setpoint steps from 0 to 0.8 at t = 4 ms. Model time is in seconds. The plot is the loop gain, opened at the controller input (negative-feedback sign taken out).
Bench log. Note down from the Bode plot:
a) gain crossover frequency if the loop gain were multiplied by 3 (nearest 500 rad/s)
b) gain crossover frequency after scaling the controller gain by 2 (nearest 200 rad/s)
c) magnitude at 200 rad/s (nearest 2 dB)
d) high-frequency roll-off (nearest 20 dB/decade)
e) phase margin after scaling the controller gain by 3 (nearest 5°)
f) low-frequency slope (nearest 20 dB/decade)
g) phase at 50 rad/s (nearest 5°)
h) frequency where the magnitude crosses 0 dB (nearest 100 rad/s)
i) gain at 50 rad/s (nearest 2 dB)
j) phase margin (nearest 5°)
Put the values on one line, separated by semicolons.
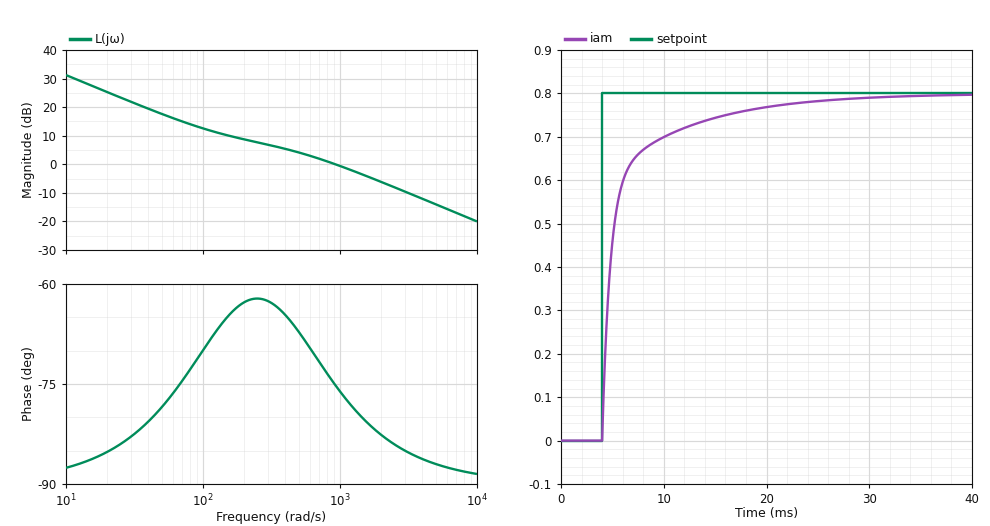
3000 rad/s; 2000 rad/s; 8 dB; -20 dB/decade; 95°; -20 dB/decade; -80°; 900 rad/s; 18 dB; 105°
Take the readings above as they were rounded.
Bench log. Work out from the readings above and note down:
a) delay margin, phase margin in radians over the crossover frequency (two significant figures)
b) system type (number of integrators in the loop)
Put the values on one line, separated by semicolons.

0.0020 s; 1
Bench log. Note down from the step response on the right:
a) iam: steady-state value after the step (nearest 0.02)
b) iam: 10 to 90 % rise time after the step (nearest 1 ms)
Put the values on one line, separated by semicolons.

0.80; 8 ms
